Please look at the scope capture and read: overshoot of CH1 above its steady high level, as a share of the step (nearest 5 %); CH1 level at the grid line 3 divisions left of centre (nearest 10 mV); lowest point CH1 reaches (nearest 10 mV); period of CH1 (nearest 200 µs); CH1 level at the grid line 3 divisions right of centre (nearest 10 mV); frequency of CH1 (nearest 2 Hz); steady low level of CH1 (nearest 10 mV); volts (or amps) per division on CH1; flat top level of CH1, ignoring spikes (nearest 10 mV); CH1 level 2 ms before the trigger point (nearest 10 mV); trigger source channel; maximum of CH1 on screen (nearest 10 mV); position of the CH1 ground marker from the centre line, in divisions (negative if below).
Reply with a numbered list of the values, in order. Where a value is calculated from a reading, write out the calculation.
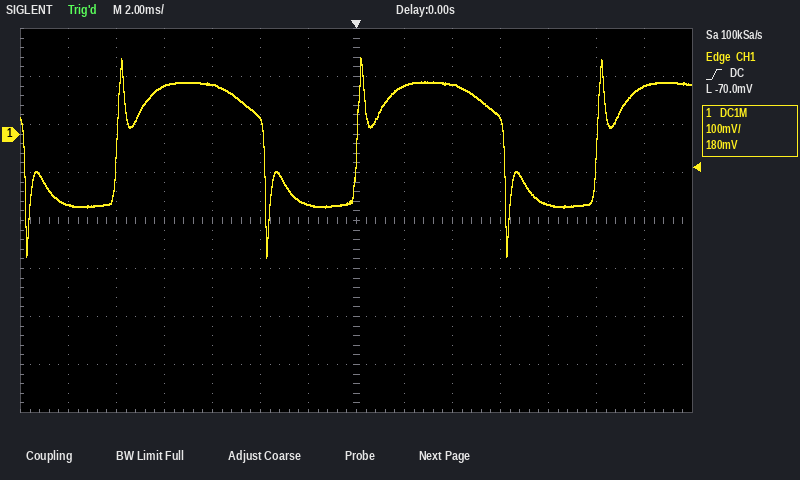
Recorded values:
1. 20 %
2. 100 mV
3. -260 mV
4. 10.0 ms
5. 30 mV
6. 1 / 10.0 ms ≈ 100 Hz
7. -150 mV
8. 100 mV
9. 110 mV
10. -150 mV
11. CH1
12. 160 mV
13. +1.8 div
